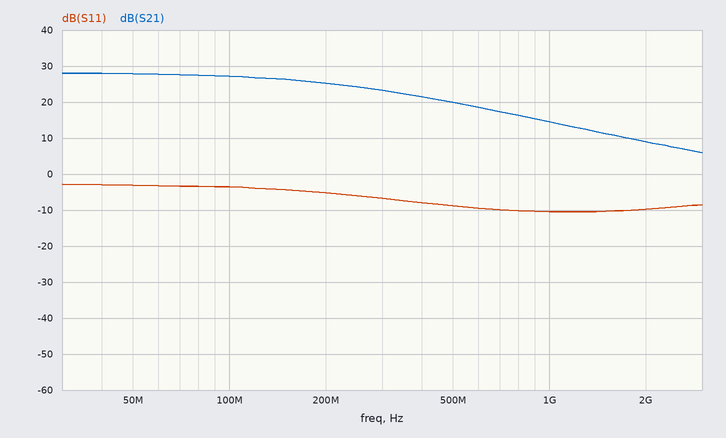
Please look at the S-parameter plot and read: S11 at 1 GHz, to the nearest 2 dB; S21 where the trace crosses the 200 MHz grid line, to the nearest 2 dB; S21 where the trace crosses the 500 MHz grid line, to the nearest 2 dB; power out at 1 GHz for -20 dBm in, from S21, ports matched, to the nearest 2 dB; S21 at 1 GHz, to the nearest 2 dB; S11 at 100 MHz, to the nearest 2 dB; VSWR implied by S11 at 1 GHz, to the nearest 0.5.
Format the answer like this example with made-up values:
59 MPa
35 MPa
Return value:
-10 dB
26 dB
20 dB
-6 dBm
14 dB
-4 dB
2.0
